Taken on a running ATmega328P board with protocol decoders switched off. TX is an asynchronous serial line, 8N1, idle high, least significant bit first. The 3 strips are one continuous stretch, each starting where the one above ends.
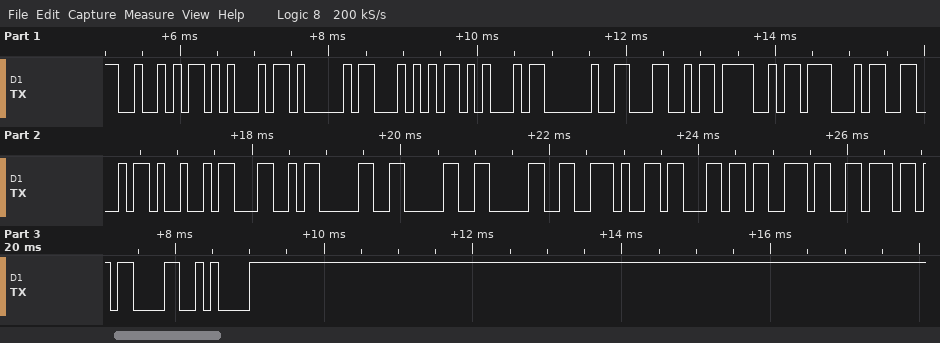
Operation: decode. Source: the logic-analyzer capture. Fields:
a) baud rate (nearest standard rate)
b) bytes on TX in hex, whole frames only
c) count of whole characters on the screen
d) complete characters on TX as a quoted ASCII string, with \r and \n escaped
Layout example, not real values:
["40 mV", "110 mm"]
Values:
["9600 baud", "52 45 41 54 45 20 4C 4F 47 46 49 4C 30 30 30 2E 63 73 76 0D 0A", "21", "\"REATE LOGFIL000.csv\\r\\n\""]
